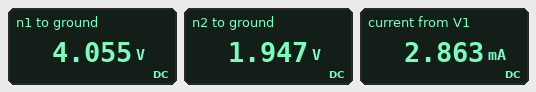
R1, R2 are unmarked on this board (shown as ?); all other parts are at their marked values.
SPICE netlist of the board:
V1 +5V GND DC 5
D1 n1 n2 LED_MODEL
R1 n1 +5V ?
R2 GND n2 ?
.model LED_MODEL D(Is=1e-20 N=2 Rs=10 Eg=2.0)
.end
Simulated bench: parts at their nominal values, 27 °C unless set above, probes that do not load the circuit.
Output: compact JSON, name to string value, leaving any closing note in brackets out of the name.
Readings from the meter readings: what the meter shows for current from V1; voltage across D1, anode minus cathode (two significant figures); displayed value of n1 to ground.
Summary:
{"what the meter shows for current from V1": "2.863 mA", "voltage across D1, anode minus cathode": "2.1 V", "displayed value of n1 to ground": "4.055 V"}
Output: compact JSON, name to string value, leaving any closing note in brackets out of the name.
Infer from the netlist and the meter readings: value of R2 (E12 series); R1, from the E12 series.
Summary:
{"value of R2": "680 Ω", "R1, from the E12 series": "330 Ω"}
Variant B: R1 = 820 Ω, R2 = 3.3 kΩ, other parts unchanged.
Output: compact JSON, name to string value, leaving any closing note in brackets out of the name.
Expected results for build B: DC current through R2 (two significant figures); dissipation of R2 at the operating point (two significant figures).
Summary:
{"DC current through R2": "720 µA", "dissipation of R2 at the operating point": "1.7 mW"}
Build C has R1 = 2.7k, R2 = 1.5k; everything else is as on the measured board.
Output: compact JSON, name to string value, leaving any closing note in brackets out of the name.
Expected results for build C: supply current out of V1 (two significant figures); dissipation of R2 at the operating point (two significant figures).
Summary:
{"supply current out of V1": "710 µA", "dissipation of R2 at the operating point": "760 µW"}
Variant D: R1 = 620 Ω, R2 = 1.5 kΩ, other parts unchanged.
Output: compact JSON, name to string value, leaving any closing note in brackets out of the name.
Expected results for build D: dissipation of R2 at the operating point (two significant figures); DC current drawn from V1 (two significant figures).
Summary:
{"dissipation of R2 at the operating point": "2.9 mW", "DC current drawn from V1": "1.4 mA"}
